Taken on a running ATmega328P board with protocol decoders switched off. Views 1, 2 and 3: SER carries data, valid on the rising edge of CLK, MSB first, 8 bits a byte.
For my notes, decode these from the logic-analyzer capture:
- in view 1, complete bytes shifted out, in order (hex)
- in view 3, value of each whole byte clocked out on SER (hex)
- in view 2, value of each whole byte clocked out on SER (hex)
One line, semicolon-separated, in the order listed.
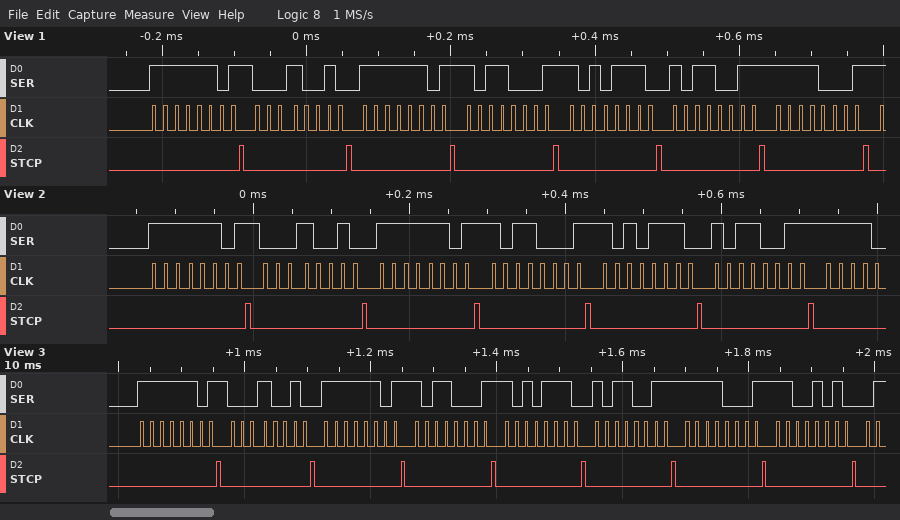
0xFD 0x12 0xFD 0xB1 0xAE 0xB3 0xF1; 0xFD 0x12 0xFD 0xB1 0xAE 0xB3 0xF1 0xCA; FD 12 FD B1 AE B3
